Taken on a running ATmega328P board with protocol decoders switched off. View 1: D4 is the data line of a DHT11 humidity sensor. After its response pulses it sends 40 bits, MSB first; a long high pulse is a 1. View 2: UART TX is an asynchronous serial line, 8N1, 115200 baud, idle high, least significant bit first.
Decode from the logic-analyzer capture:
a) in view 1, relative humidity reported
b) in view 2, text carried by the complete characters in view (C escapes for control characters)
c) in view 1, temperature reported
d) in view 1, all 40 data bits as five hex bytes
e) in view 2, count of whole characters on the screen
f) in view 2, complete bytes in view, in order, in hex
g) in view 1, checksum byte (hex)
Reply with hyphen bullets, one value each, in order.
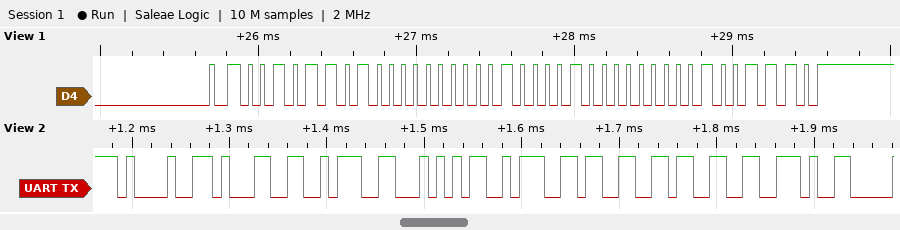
- 45 %
- "!1:T:33."
- 33.0 °C
- 2D 00 21 00 4E
- 8
- 21 31 3A 54 3A 33 33 2E
- 0x4E
